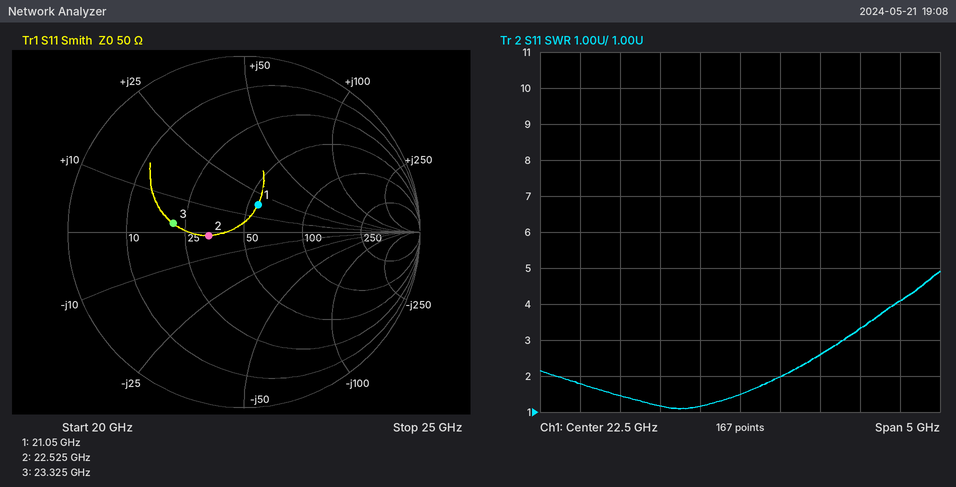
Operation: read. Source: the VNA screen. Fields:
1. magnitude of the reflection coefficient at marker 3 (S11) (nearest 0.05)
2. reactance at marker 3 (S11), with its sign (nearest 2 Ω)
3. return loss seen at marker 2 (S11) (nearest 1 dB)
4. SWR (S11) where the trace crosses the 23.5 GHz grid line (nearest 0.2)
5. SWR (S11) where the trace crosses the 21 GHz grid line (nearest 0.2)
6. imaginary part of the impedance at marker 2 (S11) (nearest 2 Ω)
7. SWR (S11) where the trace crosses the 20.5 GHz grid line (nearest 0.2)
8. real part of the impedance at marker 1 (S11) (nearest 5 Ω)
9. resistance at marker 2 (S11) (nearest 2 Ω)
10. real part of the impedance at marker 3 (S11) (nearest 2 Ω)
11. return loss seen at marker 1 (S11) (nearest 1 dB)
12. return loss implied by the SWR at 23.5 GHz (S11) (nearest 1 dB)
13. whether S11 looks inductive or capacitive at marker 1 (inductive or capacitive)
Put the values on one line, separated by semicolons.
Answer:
0.40; +2 Ω; 14 dB; 2.6; 1.4; -2 Ω; 1.8; 55 Ω; 34 Ω; 22 Ω; 15 dB; 7 dB; inductive
